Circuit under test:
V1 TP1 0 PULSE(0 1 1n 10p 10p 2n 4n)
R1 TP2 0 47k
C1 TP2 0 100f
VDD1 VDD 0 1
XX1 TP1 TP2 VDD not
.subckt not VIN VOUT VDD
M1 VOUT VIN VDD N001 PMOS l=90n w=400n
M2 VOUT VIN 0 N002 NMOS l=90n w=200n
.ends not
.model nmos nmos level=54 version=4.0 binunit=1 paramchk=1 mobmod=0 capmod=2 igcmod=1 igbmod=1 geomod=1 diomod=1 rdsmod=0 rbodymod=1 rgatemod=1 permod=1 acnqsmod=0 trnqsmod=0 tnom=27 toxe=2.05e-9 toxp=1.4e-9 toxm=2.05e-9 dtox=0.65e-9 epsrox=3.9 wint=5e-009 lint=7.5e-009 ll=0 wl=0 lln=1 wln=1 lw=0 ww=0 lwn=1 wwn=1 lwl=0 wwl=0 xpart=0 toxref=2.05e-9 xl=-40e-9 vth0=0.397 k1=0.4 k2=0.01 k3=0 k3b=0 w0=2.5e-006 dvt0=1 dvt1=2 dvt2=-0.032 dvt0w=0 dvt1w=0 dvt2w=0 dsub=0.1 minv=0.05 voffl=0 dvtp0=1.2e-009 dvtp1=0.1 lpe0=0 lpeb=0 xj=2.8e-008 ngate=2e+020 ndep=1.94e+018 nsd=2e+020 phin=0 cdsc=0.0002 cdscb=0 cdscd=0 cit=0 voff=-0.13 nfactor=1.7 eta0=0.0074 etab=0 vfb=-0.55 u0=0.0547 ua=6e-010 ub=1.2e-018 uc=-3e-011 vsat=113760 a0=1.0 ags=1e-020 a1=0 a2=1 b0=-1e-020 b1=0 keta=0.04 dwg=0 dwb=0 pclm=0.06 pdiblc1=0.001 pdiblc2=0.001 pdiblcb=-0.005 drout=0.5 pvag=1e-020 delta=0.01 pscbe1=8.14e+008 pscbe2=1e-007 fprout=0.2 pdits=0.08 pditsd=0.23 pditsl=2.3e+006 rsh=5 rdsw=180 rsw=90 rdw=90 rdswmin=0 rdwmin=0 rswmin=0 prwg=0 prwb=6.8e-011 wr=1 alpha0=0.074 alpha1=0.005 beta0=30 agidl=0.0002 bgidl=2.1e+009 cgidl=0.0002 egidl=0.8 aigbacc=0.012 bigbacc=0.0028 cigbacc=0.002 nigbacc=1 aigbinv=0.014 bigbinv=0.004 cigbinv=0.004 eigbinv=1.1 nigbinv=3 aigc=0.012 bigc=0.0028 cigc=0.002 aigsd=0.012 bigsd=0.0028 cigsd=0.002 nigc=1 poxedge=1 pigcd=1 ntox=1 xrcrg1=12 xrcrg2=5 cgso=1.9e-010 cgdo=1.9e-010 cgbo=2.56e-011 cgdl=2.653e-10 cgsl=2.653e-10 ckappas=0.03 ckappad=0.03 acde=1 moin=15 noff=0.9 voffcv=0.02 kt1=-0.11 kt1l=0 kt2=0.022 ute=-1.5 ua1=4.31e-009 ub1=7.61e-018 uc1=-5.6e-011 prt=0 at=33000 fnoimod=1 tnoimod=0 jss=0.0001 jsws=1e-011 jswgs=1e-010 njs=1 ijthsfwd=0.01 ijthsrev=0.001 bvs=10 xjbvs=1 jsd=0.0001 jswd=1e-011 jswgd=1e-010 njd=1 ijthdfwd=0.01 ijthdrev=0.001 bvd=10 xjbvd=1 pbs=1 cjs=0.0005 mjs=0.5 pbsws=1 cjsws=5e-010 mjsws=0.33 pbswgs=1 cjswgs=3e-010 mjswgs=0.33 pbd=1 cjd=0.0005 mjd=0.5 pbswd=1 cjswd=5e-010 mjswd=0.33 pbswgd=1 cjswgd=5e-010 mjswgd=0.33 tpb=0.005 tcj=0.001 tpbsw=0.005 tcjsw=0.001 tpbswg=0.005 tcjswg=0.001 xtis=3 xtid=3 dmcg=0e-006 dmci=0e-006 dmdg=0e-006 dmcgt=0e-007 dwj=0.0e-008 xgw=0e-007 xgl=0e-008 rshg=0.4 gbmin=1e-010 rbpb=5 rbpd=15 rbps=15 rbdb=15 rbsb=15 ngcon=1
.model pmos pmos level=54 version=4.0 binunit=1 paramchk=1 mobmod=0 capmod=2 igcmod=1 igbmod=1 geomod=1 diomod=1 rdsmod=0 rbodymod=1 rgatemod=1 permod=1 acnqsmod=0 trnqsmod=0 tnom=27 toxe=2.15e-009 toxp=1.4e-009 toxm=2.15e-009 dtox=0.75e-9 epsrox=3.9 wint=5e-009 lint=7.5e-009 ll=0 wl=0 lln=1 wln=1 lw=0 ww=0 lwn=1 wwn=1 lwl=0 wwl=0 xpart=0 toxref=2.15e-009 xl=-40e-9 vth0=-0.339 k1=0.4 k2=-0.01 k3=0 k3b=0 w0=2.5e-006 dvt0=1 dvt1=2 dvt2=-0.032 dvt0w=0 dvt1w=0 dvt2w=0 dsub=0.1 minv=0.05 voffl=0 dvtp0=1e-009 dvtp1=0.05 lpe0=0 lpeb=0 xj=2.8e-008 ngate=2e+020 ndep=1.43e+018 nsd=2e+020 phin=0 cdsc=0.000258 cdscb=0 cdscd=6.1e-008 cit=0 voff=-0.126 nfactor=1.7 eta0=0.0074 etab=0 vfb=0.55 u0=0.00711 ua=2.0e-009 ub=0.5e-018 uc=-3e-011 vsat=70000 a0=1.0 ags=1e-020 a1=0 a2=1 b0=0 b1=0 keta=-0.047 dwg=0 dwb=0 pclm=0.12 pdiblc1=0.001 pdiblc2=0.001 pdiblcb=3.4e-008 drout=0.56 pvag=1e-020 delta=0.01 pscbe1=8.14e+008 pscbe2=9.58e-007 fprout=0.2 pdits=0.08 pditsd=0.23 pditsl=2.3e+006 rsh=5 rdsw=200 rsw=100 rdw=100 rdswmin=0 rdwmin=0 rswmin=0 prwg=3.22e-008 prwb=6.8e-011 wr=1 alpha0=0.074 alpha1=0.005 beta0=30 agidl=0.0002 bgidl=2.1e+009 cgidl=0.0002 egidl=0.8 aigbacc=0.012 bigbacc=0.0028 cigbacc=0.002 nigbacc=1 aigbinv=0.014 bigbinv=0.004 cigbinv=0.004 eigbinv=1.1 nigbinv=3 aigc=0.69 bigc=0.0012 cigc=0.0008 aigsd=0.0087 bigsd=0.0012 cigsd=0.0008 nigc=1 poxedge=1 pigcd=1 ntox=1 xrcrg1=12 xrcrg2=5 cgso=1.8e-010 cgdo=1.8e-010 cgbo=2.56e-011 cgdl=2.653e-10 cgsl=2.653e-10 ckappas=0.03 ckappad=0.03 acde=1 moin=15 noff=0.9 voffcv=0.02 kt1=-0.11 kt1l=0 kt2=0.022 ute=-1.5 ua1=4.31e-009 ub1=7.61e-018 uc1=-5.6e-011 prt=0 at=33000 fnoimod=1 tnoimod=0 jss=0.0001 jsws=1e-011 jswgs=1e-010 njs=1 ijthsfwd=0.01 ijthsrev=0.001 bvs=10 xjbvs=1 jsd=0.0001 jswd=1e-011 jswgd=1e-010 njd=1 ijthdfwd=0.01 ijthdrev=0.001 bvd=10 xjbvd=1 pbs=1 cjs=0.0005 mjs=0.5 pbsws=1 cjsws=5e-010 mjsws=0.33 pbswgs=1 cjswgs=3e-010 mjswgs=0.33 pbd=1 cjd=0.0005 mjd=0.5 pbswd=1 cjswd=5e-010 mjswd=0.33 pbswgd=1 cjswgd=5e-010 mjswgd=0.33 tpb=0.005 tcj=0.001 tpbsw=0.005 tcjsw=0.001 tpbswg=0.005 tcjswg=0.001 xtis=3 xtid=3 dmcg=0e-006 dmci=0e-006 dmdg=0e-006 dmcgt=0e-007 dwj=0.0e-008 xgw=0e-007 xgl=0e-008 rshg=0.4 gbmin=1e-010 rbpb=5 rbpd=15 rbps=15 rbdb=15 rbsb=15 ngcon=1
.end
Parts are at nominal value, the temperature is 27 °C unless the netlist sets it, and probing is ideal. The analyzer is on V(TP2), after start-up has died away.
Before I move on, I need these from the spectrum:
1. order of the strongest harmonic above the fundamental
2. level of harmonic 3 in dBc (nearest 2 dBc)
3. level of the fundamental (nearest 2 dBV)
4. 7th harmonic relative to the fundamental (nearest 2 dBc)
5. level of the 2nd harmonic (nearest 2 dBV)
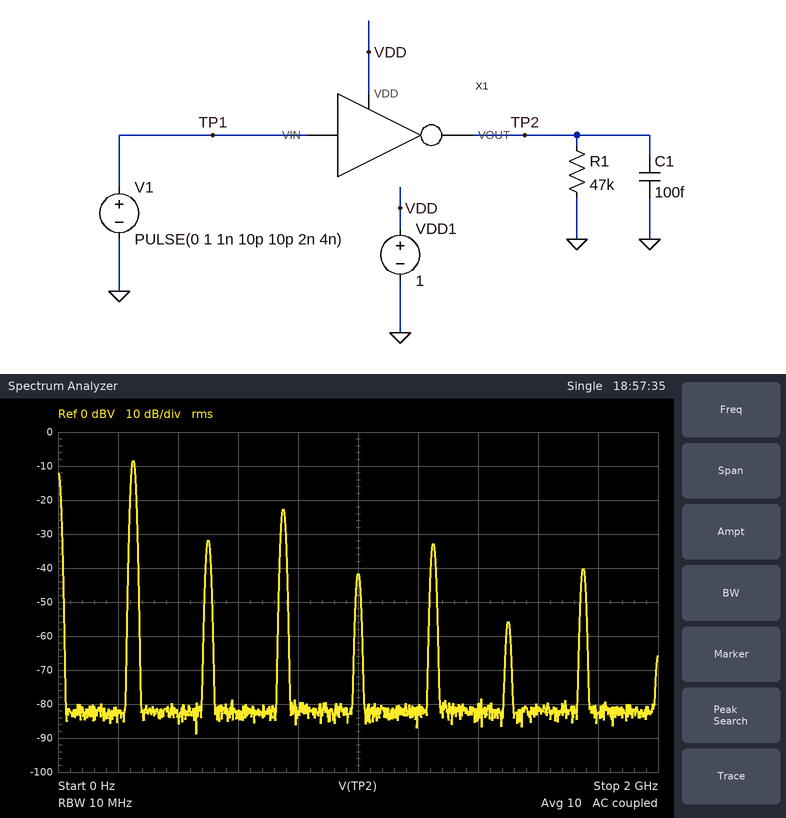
3
-14 dBc
-8 dBV
-32 dBc
-32 dBV
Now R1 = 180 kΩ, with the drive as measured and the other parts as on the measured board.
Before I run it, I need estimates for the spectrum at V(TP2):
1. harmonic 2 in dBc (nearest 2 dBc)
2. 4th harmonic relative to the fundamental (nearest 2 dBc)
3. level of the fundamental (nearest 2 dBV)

-26 dBc
-36 dBc
-8 dBV
